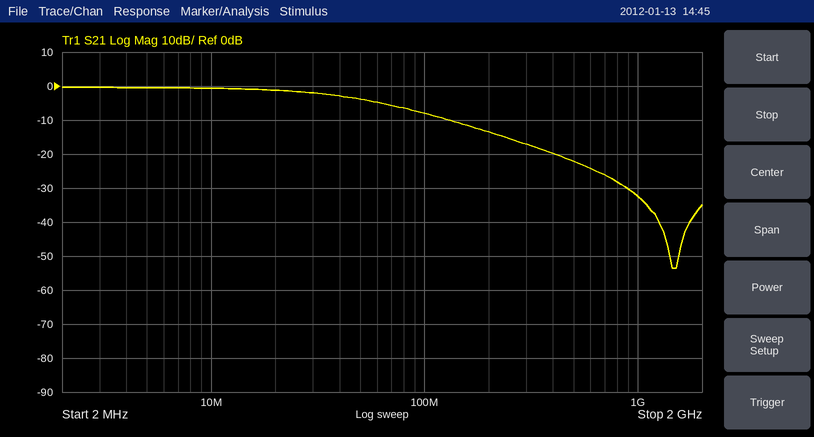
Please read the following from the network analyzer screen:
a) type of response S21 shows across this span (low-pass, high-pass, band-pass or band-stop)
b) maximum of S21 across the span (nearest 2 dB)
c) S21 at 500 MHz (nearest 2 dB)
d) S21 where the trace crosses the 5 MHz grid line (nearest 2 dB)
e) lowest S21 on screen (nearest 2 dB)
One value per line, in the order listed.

low-pass
0 dB
-22 dB
0 dB
-54 dB
